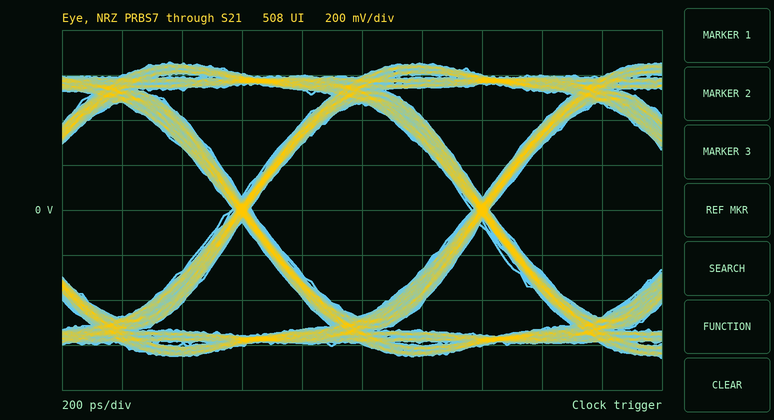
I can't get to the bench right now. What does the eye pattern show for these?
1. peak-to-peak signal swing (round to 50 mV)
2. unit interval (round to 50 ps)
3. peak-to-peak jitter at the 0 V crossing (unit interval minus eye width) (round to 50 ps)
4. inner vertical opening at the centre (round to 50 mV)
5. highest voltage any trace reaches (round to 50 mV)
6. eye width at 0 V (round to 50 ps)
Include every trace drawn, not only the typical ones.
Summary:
1.30 V
800 ps
50 ps
950 mV
650 mV
750 ps
